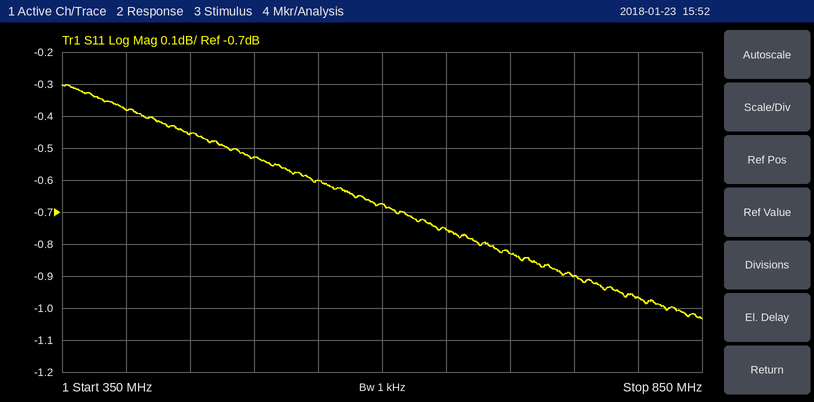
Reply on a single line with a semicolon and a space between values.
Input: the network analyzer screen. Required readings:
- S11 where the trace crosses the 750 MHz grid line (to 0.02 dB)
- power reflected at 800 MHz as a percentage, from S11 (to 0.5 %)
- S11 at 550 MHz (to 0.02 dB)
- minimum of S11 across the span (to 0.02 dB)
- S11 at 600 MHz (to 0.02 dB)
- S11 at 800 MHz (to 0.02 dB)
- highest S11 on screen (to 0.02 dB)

-0.90 dB; 80.0 %; -0.60 dB; -1.04 dB; -0.68 dB; -0.96 dB; -0.30 dB
